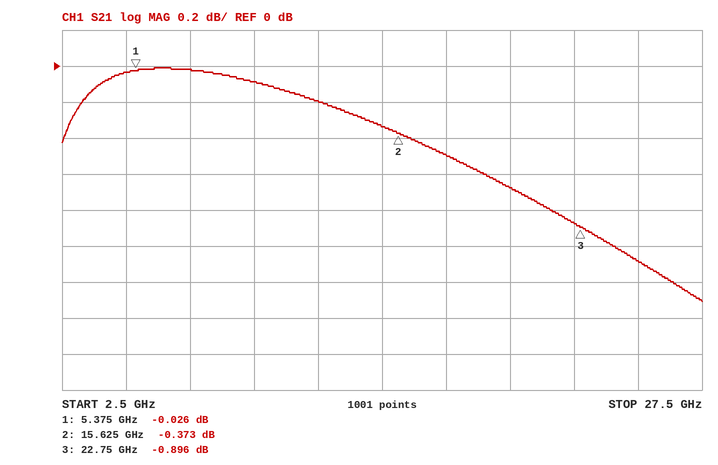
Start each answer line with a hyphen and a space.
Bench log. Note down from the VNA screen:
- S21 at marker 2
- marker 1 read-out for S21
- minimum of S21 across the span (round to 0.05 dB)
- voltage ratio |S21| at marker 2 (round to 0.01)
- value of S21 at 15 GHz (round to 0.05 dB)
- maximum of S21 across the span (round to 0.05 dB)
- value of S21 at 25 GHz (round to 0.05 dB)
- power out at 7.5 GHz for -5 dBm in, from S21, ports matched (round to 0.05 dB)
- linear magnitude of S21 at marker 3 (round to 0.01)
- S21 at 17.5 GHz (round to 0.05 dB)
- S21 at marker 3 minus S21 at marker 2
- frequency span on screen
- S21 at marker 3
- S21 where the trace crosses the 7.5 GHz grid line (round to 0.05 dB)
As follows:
- -0.373 dB
- -0.026 dB
- -1.30 dB
- 0.96
- -0.35 dB
- 0.00 dB
- -1.10 dB
- -5.00 dBm
- 0.90
- -0.50 dB
- -0.523 dB
- 25 GHz
- -0.896 dB
- 0.00 dB
